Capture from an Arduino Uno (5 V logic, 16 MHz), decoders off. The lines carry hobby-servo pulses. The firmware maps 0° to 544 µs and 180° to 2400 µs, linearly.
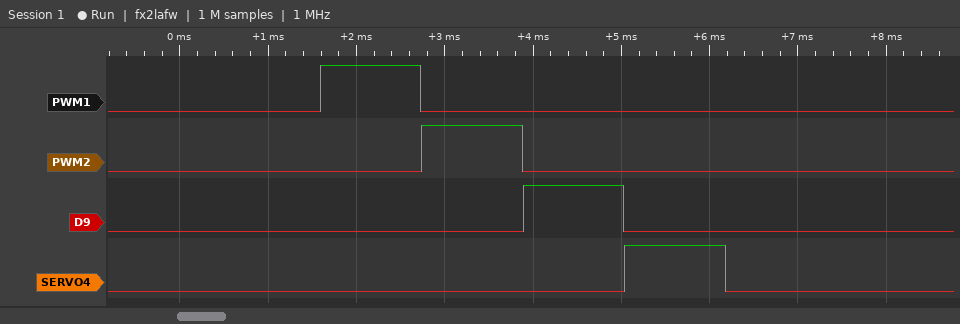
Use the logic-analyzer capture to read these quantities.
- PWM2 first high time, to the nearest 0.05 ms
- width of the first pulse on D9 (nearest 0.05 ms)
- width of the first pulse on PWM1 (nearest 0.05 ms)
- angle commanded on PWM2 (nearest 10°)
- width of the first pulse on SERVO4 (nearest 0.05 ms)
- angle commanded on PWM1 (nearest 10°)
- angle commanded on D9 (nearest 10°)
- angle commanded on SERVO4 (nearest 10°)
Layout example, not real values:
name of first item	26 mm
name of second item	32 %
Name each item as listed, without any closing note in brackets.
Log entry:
PWM2 first high time, to the nearest 0.05 ms	1.15 ms
width of the first pulse on D9	1.15 ms
width of the first pulse on PWM1	1.15 ms
angle commanded on PWM2	60°
width of the first pulse on SERVO4	1.15 ms
angle commanded on PWM1	60°
angle commanded on D9	60°
angle commanded on SERVO4	60°
